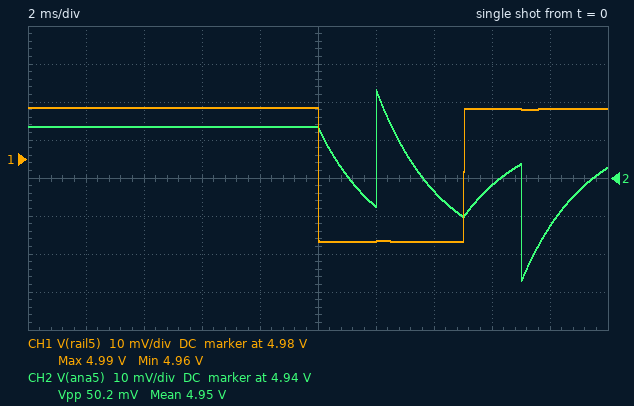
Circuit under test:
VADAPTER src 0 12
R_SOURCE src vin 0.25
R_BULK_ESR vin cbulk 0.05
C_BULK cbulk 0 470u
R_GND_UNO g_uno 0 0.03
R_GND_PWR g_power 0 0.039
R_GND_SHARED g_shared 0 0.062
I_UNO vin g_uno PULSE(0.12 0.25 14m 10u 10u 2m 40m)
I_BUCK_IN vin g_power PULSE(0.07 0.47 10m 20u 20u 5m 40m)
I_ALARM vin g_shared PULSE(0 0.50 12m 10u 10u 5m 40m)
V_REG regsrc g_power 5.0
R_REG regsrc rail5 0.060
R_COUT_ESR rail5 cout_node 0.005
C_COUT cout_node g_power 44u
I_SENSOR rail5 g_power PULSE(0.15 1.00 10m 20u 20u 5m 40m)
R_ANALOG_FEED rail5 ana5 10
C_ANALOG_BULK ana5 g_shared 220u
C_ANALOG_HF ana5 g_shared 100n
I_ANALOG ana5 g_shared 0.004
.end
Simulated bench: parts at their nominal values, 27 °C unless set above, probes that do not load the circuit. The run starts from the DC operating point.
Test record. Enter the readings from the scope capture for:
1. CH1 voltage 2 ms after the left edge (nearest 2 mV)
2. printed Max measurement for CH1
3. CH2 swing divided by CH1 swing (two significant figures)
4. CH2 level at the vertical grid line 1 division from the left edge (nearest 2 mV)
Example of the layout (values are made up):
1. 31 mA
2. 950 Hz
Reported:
1. 4.994 V
2. 4.99 V
3. 1.4
4. 4.954 V
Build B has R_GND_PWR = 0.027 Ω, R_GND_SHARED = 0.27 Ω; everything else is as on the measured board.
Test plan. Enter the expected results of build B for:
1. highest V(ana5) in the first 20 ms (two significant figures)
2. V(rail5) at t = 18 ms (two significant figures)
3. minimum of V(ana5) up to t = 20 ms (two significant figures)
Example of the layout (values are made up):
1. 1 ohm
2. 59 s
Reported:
1. 5.1 V
2. 5.0 V
3. 4.8 V
